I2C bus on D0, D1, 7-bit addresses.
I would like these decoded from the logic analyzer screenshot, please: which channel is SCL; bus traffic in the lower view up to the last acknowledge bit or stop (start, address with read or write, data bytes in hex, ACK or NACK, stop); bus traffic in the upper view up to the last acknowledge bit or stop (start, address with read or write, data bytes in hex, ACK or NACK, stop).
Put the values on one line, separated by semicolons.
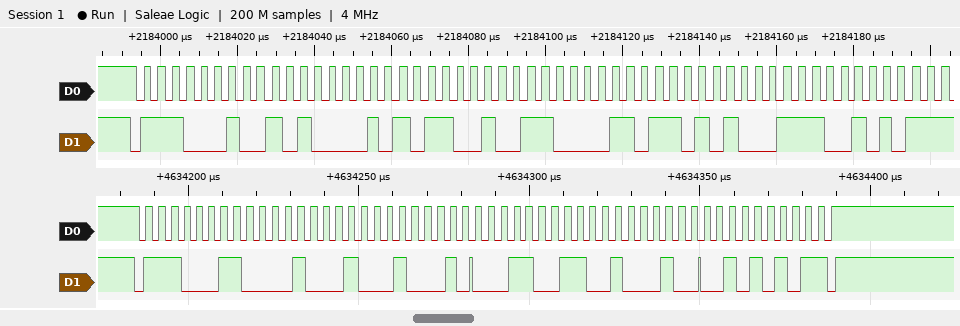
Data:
D0; start, address 71 read ACK, 11 ACK, 22 ACK, 33 ACK, 44 ACK, 55 NACK, stop; start, address 71 write ACK, A1 ACK, B2 ACK, C3 ACK, D4 ACK, E5 ACK
